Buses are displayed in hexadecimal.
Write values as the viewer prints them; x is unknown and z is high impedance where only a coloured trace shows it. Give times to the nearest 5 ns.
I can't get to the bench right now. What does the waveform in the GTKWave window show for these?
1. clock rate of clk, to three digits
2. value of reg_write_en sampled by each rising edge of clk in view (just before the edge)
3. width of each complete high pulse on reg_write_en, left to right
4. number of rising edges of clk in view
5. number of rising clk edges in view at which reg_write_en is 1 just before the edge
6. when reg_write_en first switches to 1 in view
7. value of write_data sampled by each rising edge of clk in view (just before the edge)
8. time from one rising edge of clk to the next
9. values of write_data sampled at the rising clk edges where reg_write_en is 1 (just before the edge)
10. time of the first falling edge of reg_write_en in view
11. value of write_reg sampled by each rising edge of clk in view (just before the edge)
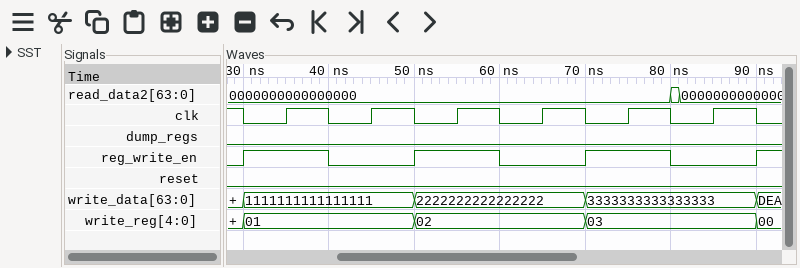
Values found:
100 MHz
1 0 1 0 1 0
10 ns, 10 ns, 10 ns
6
3
30 ns
1111111111111111, 1111111111111111, 2222222222222222, 2222222222222222, 3333333333333333, 3333333333333333
10 ns
1111111111111111, 2222222222222222, 3333333333333333
40 ns
01, 01, 02, 02, 03, 03
